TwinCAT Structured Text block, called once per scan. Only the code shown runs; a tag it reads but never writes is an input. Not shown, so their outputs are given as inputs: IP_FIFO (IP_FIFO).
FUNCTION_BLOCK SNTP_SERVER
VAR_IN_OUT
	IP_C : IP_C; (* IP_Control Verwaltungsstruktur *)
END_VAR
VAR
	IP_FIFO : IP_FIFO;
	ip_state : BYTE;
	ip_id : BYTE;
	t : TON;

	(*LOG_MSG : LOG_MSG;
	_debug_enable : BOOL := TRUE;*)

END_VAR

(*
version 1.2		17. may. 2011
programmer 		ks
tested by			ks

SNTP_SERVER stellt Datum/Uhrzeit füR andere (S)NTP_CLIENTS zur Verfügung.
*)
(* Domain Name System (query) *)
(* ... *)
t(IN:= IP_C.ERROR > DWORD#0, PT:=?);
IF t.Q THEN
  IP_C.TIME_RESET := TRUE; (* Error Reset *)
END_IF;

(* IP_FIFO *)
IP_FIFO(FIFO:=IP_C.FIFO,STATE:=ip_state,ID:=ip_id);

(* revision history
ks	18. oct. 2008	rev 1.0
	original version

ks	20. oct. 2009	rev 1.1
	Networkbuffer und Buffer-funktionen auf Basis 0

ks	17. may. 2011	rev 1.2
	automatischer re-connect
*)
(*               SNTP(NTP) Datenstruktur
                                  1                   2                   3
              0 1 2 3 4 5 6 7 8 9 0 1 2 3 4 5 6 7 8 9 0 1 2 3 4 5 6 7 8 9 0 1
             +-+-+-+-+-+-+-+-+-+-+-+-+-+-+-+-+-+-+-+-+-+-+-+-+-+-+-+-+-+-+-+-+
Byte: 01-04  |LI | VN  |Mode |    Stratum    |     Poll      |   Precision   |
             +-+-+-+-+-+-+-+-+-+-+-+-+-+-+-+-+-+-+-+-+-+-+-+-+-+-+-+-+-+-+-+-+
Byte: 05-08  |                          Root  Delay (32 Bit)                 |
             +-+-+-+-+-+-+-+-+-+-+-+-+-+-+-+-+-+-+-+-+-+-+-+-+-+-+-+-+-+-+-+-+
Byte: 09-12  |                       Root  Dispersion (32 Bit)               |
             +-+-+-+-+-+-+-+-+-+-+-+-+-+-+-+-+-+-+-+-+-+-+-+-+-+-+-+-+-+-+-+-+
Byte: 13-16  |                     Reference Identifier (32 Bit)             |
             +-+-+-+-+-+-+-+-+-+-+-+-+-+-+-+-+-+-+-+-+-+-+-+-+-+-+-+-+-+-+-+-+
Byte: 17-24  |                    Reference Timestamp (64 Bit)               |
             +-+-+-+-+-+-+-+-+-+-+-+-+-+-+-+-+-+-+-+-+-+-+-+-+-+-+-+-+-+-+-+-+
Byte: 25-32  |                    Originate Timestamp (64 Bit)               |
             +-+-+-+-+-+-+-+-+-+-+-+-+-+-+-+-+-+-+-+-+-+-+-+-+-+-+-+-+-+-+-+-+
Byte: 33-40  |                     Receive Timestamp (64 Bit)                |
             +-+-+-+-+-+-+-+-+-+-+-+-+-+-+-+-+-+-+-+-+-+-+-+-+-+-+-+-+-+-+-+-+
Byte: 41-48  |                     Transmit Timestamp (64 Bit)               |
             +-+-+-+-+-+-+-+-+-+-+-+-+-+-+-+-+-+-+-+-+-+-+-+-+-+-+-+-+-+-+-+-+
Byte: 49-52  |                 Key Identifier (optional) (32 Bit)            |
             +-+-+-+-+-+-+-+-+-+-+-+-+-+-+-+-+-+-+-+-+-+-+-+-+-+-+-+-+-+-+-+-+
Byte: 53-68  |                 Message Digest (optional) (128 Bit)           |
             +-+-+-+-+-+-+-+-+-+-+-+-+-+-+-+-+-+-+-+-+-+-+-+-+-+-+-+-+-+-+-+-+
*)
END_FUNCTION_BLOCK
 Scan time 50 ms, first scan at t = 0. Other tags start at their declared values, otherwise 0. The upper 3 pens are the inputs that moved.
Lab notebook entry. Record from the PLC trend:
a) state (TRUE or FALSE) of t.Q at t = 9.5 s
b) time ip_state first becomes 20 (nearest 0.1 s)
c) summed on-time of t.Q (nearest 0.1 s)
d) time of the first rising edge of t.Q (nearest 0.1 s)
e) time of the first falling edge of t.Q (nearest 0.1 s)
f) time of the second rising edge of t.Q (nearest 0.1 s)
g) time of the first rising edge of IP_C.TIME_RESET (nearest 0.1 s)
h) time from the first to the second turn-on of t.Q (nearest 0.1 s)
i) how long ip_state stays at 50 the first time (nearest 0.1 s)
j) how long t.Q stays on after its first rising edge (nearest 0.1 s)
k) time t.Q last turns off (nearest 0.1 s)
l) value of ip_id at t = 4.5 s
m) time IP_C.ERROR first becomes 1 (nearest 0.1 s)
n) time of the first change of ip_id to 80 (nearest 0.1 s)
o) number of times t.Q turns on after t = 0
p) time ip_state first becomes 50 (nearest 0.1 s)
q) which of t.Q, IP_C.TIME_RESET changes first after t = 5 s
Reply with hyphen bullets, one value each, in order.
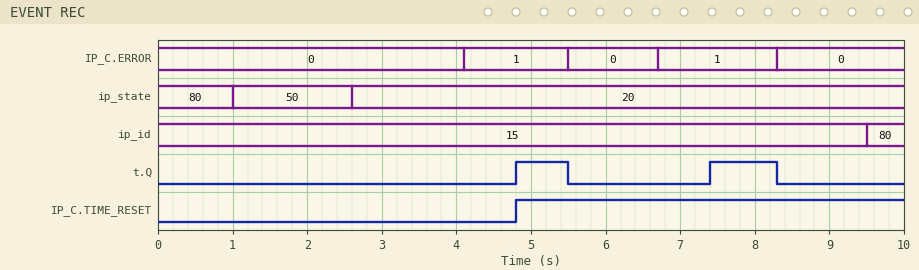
- FALSE
- 2.6 s
- 1.6 s
- 4.8 s
- 5.5 s
- 7.4 s
- 4.8 s
- 2.6 s
- 1.6 s
- 0.7 s
- 8.3 s
- 15
- 4.1 s
- 9.5 s
- 2
- 1.0 s
- t.Q
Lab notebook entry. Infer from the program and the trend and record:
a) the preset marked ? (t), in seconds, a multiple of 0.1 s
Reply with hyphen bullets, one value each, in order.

- 0.7 s
